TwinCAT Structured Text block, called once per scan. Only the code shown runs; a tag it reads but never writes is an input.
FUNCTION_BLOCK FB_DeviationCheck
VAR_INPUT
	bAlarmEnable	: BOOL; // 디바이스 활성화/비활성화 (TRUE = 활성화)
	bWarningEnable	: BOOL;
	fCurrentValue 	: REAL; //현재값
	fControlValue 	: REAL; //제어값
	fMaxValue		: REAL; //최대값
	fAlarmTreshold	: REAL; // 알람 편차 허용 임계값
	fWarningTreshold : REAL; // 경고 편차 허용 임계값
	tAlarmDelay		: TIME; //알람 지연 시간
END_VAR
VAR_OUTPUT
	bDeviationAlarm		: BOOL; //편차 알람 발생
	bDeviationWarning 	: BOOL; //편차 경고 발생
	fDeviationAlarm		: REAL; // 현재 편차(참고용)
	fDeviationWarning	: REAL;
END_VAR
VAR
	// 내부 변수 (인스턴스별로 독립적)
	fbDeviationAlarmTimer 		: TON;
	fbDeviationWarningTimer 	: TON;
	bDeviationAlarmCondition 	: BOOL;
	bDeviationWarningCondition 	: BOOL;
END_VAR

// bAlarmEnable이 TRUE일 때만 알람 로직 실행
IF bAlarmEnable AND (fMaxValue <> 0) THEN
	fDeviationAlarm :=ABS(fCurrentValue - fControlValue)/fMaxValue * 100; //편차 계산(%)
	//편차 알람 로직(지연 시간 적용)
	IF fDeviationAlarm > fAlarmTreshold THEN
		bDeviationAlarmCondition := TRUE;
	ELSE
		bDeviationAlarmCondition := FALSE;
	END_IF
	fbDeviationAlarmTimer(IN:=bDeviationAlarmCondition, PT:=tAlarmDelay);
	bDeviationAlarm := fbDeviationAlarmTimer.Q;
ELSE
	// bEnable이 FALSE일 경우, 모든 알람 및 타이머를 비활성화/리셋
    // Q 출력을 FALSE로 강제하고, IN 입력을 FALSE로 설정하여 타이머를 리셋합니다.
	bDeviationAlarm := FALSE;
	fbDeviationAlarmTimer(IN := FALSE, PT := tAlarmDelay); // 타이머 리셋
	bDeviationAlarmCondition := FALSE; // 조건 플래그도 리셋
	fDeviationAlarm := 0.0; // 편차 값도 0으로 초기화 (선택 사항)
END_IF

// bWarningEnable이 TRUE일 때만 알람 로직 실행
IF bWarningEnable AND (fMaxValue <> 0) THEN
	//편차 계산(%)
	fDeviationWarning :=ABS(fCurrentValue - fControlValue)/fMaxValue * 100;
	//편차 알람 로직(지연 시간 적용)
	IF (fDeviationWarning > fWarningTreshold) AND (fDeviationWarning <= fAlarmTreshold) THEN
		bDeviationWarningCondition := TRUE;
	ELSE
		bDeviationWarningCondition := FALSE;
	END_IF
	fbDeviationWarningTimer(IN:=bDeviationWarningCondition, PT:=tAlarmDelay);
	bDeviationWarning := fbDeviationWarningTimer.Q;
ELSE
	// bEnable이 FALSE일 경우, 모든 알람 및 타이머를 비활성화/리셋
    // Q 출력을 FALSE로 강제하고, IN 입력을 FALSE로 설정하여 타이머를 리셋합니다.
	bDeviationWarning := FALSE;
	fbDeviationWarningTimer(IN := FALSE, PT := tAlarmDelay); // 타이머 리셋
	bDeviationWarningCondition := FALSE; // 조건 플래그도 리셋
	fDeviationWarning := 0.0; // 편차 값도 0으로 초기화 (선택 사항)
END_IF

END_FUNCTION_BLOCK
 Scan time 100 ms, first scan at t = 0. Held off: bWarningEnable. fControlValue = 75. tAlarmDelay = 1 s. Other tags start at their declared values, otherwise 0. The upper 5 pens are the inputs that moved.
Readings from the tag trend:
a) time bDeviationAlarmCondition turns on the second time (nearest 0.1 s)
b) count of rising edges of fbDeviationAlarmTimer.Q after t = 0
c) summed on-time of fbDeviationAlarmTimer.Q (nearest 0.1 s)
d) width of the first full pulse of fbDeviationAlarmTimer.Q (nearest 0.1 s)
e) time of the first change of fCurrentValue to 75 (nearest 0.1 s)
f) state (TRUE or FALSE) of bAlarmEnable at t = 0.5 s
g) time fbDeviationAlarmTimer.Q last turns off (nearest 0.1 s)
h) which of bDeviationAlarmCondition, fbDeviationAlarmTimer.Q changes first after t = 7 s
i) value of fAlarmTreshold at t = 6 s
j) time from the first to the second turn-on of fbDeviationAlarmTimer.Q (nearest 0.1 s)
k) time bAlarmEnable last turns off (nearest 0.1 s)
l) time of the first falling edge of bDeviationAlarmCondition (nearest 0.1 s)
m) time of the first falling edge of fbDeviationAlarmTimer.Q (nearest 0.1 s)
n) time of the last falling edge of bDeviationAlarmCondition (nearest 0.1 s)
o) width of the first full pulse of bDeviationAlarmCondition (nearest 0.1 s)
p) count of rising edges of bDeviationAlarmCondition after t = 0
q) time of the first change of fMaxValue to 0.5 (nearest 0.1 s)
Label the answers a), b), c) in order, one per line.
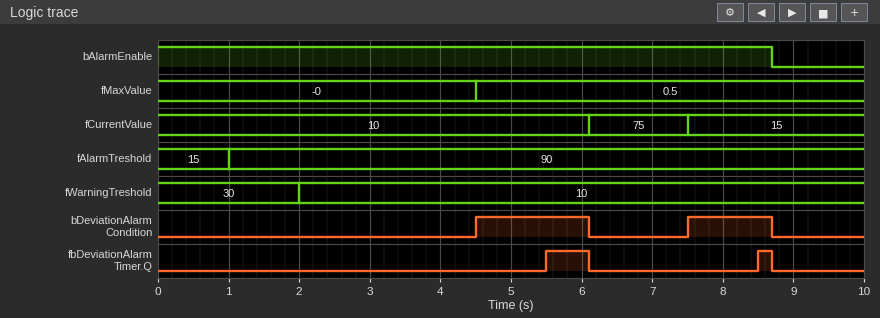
a) 7.5 s
b) 2
c) 0.8 s
d) 0.6 s
e) 6.1 s
f) TRUE
g) 8.7 s
h) bDeviationAlarmCondition
i) 90
j) 3.0 s
k) 8.7 s
l) 6.1 s
m) 6.1 s
n) 8.7 s
o) 1.6 s
p) 2
q) 4.5 s
